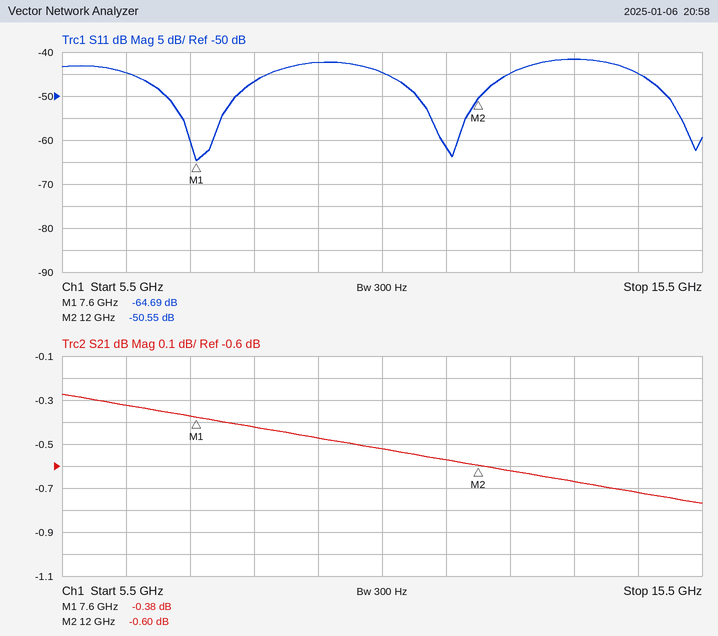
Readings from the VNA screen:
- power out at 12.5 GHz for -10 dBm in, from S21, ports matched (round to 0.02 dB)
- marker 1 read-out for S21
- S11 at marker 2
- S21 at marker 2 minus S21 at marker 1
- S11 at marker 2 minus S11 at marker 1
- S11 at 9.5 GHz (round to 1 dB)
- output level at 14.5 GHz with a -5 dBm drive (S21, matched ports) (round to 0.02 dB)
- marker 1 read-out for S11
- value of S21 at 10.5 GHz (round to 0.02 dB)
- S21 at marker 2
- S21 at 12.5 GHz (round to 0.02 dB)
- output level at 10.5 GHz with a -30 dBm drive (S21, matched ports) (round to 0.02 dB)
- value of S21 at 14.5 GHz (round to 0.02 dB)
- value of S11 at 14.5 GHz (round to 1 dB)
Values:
-10.62 dBm
-0.38 dB
-50.55 dB
-0.22 dB
14.14 dB
-42 dB
-5.72 dBm
-64.69 dB
-0.52 dB
-0.60 dB
-0.62 dB
-30.52 dBm
-0.72 dB
-45 dB
